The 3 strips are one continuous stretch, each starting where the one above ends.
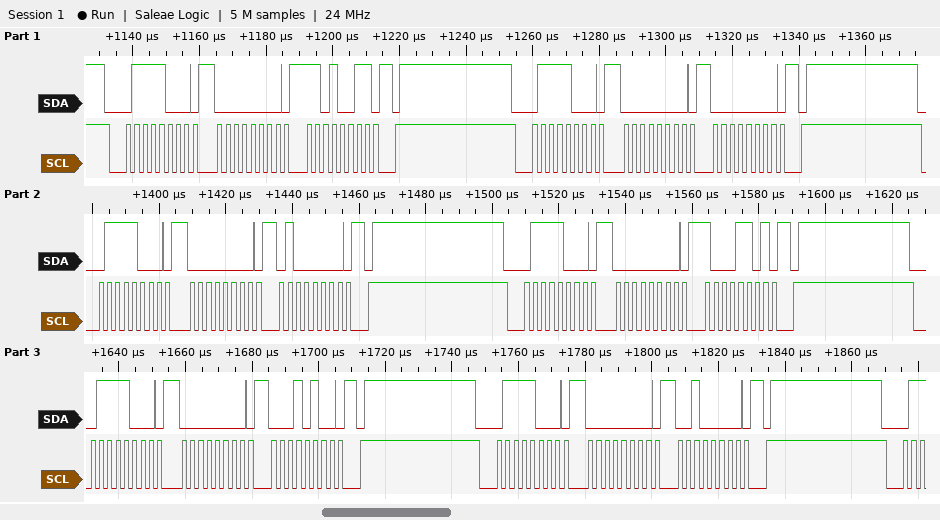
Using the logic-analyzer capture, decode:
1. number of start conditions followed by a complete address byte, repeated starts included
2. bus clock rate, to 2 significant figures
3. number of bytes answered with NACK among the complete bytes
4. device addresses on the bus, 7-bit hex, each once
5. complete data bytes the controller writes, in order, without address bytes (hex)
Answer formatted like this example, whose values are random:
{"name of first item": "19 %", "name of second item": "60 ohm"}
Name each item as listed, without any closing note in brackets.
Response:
{"number of start conditions followed by a complete address byte, repeated starts included": "6", "bus clock rate, to 2 significant figures": "400 kHz", "number of bytes answered with NACK among the complete bytes": "0", "device addresses on the bus, 7-bit hex, each once": "0x3C", "complete data bytes the controller writes, in order, without address bytes": "00 D3 00 00 00 40 00 8D 00 14 00 20"}
